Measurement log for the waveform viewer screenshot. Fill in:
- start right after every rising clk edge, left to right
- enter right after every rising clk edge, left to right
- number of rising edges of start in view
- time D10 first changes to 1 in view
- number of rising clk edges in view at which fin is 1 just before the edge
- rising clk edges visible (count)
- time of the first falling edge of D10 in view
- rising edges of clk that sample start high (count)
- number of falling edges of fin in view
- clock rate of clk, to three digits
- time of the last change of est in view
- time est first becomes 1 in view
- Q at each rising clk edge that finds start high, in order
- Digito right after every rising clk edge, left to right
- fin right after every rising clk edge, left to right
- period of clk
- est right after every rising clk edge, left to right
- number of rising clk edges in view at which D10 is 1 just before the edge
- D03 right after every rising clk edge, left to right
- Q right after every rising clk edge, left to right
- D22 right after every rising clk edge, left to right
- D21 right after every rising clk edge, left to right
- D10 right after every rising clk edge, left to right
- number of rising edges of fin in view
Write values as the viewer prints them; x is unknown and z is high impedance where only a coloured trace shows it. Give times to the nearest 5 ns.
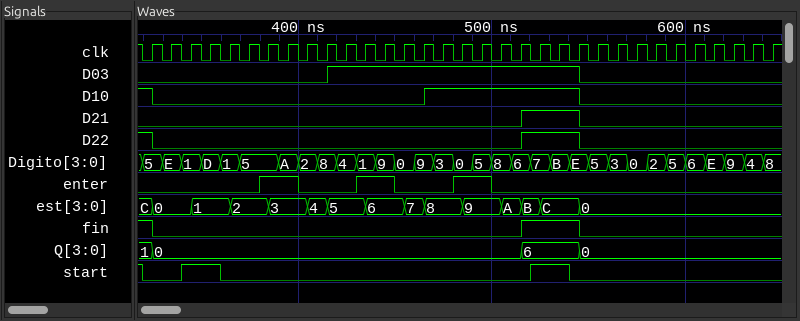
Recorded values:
0 0 1 1 0 0 0 0 0 0 0 0 0 0 0 0 0 0 0 0 1 1 0 0 0 0 0 0 0 0 0 0 0
0 0 0 0 0 0 1 1 0 0 0 1 1 0 0 0 1 1 0 0 0 0 0 0 0 0 0 0 0 0 0 0 0
2
465 ns
4
33
325 ns
4
2
100 MHz
545 ns
345 ns
0, 0, 6, 6
5, E, 1, D, 1, 5, 5, A, 2, 8, 4, 1, 9, 0, 9, 3, 0, 5, 8, 6, 7, B, E, 5, 3, 0, 2, 5, 6, E, 9, 4, 8
0 0 0 0 0 0 0 0 0 0 0 0 0 0 0 0 0 0 0 1 1 1 0 0 0 0 0 0 0 0 0 0 0
10 ns
0, 0, 1, 1, 2, 2, 3, 3, 4, 5, 5, 6, 6, 7, 8, 8, 9, 9, A, B, C, C, 0, 0, 0, 0, 0, 0, 0, 0, 0, 0, 0
9
0 0 0 0 0 0 0 0 0 1 1 1 1 1 1 1 1 1 1 1 1 1 0 0 0 0 0 0 0 0 0 0 0
0, 0, 0, 0, 0, 0, 0, 0, 0, 0, 0, 0, 0, 0, 0, 0, 0, 0, 0, 6, 6, 6, 0, 0, 0, 0, 0, 0, 0, 0, 0, 0, 0
0 0 0 0 0 0 0 0 0 0 0 0 0 0 0 0 0 0 0 1 1 1 0 0 0 0 0 0 0 0 0 0 0
0 0 0 0 0 0 0 0 0 0 0 0 0 0 0 0 0 0 0 1 1 1 0 0 0 0 0 0 0 0 0 0 0
0 0 0 0 0 0 0 0 0 0 0 0 0 0 1 1 1 1 1 1 1 1 0 0 0 0 0 0 0 0 0 0 0
1
